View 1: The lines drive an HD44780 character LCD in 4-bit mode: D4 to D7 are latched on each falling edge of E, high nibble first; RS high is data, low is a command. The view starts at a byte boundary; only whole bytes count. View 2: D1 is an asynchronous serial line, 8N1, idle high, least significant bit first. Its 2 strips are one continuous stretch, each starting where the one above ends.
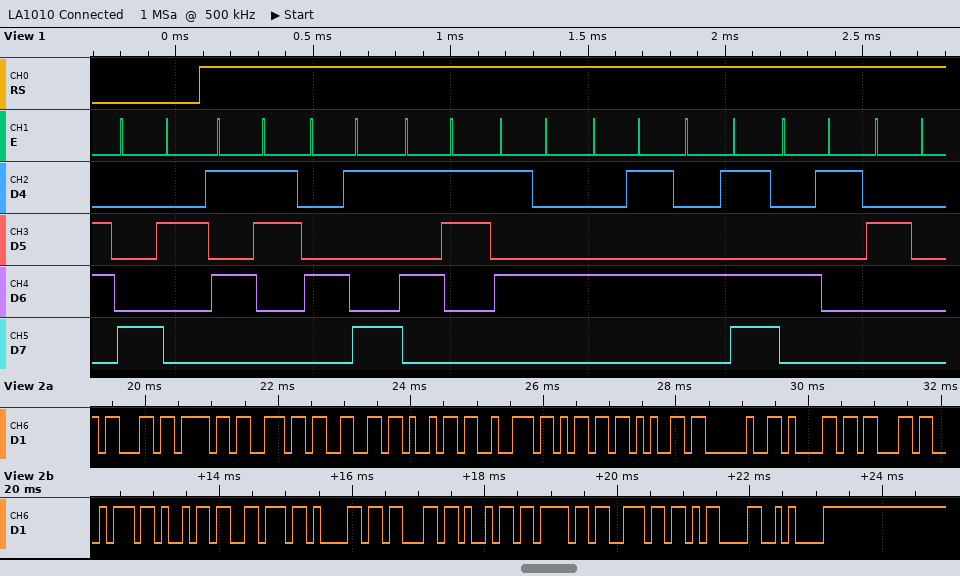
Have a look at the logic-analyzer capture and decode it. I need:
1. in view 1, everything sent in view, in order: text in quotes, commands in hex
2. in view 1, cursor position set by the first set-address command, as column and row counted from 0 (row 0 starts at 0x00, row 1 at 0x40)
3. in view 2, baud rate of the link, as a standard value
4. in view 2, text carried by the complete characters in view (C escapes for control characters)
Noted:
0x82 "SISTEMA "
column 2, row 0
9600 baud
"confirme activacion\r\n"
